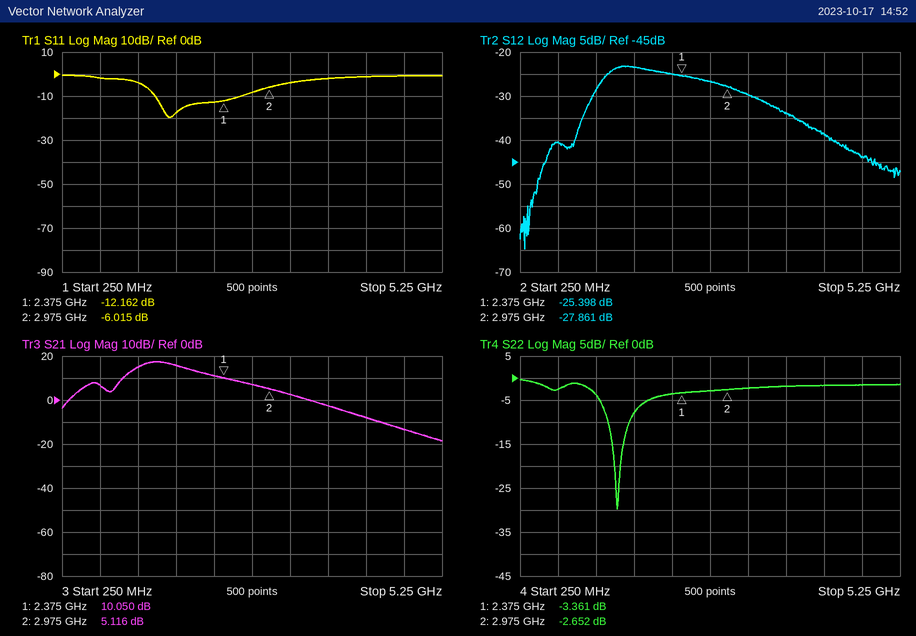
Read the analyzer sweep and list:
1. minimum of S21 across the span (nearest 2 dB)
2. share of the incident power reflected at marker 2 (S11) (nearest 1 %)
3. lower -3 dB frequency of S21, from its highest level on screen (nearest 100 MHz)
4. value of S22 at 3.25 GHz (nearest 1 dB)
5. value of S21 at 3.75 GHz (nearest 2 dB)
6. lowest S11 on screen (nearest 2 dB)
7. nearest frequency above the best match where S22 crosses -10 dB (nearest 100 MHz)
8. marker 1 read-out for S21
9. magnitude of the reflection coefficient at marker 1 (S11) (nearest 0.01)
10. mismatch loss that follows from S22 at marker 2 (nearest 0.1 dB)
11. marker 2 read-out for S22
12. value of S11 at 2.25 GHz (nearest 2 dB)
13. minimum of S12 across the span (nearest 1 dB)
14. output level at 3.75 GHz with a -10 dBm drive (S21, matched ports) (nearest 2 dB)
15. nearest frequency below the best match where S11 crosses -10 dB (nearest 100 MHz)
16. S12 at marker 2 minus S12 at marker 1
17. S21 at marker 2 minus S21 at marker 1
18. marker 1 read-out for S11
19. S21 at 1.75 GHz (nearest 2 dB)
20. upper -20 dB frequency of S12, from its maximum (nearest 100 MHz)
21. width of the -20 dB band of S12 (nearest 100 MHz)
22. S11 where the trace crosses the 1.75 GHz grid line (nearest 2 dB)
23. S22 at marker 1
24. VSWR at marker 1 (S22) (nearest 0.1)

-18 dB
25 %
1.2 GHz
-2 dB
-2 dB
-20 dB
1.7 GHz
10.050 dB
0.25
3.4 dB
-2.652 dB
-12 dB
-65 dB
-12 dBm
1.5 GHz
-2.463 dB
-4.934 dB
-12.162 dB
16 dB
4.7 GHz
4.1 GHz
-18 dB
-3.361 dB
5.2
